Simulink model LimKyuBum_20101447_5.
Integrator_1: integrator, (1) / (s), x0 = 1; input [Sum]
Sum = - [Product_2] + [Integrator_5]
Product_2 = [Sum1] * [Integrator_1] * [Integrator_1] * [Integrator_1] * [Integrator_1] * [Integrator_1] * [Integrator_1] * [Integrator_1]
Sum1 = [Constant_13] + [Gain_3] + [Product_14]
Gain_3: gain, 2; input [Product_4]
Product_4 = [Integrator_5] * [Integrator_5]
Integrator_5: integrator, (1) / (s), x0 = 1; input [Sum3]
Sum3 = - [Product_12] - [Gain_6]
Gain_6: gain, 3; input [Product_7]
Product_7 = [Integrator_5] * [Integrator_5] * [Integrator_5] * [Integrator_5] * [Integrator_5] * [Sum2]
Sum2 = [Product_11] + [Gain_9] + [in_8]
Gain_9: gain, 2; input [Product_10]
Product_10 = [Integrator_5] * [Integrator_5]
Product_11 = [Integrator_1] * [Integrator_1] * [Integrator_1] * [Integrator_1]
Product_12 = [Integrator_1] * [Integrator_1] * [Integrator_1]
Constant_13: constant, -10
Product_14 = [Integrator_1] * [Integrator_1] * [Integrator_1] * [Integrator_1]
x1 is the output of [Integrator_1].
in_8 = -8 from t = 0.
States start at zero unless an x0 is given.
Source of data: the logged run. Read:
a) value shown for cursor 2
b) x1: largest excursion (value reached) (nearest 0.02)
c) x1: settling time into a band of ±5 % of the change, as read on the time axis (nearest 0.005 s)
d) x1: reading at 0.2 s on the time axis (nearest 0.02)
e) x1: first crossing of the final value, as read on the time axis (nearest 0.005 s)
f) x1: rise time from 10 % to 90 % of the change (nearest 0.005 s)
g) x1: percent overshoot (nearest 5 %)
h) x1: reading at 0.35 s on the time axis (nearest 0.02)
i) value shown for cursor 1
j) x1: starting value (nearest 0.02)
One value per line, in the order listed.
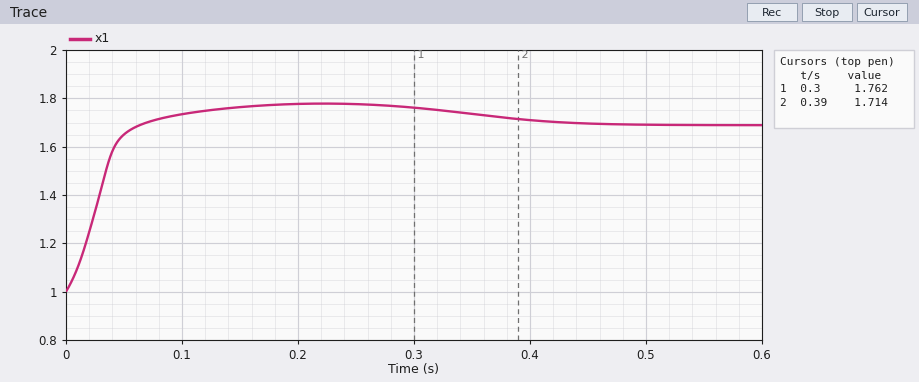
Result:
1.714
1.78
0.370 s
1.78
0.065 s
0.035 s
15 %
1.74
1.762
1.00
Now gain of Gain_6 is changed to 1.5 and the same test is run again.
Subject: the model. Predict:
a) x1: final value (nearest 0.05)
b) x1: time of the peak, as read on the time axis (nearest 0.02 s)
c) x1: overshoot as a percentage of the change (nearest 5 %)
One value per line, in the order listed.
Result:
1.65
0.22 s
20 %
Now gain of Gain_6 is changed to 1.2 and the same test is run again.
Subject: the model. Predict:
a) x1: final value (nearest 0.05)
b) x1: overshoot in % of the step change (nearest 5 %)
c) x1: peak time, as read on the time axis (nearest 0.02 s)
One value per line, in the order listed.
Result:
1.65
20 %
0.22 s
